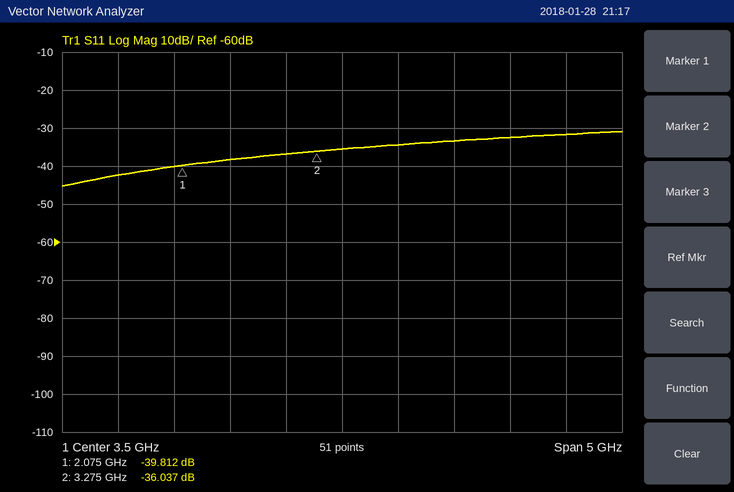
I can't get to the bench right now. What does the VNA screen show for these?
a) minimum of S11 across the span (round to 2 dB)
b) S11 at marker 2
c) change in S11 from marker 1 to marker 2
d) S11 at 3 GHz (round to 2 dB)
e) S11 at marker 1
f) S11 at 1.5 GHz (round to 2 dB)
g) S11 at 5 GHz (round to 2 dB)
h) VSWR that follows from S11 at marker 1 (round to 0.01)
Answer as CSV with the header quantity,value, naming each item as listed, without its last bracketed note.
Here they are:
quantity,value
minimum of S11 across the span,-46 dB
S11 at marker 2,-36.037 dB
change in S11 from marker 1 to marker 2,3.775 dB
S11 at 3 GHz,-36 dB
S11 at marker 1,-39.812 dB
S11 at 1.5 GHz,-42 dB
S11 at 5 GHz,-32 dB
VSWR that follows from S11 at marker 1,1.02
